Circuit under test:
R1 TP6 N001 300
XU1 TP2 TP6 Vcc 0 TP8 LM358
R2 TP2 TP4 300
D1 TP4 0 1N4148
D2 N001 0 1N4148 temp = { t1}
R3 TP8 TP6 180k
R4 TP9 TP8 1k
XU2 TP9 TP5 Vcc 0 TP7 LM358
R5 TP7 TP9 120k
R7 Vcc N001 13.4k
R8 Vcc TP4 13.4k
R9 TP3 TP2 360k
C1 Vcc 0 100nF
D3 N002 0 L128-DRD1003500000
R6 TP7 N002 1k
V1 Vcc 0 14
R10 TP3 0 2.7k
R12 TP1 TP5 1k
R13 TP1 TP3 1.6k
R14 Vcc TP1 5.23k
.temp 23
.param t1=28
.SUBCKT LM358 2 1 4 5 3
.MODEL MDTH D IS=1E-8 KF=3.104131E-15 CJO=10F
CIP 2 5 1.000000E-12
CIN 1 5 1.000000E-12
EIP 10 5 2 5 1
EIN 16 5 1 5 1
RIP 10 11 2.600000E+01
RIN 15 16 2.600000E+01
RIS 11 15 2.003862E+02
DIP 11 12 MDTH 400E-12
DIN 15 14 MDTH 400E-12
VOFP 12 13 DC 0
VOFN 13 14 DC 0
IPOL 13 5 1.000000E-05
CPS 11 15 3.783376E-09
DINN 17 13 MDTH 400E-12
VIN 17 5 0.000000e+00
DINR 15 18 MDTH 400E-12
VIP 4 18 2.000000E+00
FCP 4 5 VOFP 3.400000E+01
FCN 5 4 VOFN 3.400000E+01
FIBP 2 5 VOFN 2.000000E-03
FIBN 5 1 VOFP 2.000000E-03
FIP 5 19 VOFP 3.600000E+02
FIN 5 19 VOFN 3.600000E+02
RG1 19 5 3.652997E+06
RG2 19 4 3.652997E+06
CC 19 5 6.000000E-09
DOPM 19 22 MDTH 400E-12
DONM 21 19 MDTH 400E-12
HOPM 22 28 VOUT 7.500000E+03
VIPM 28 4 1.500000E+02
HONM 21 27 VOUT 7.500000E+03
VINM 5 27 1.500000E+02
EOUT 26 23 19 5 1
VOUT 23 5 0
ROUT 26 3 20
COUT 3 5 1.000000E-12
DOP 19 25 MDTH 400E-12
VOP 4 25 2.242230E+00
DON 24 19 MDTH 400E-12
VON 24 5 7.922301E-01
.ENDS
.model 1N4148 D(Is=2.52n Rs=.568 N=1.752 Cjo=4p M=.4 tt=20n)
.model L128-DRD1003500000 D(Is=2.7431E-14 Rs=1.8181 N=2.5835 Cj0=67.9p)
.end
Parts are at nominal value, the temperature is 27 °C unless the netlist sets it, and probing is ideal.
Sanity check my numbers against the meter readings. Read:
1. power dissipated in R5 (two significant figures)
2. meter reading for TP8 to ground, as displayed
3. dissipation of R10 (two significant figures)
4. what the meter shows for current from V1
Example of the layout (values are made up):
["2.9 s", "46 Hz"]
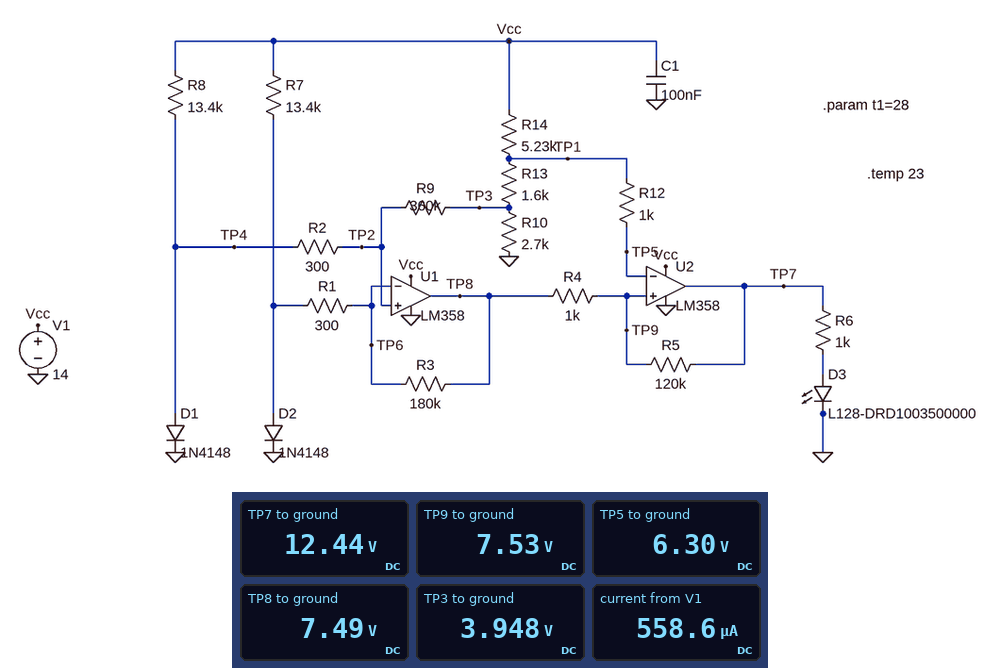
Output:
["200 µW", "7.49 V", "5.8 mW", "558.6 µA"]
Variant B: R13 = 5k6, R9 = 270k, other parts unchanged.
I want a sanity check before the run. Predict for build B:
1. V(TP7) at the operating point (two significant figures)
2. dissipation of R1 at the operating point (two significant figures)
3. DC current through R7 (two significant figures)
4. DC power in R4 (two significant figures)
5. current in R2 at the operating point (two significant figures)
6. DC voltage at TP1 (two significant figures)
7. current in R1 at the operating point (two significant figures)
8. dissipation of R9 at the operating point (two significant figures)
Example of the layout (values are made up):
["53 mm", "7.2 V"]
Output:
["-100 mV", "410 nW", "1.0 mA", "3.7 µW", "8.1 µA", "8.6 V", "37 µA", "18 µW"]
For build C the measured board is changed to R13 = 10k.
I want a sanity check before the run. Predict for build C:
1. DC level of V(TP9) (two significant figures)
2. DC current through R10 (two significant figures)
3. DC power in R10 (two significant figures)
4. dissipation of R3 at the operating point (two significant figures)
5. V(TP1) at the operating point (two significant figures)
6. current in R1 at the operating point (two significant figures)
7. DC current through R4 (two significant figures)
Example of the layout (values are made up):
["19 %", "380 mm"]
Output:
["6.5 V", "780 µA", "1.6 mW", "200 µW", "9.9 V", "33 µA", "55 µA"]
